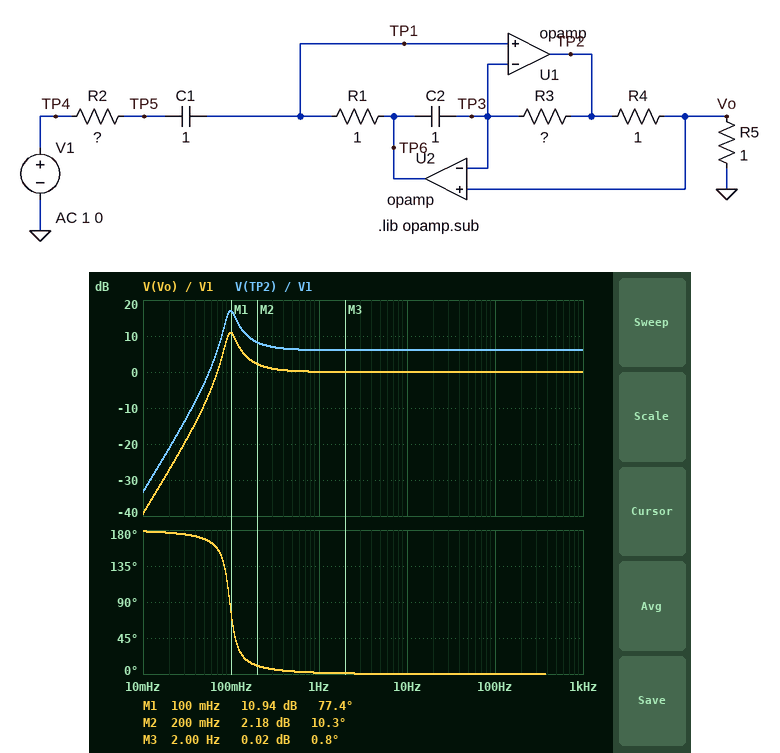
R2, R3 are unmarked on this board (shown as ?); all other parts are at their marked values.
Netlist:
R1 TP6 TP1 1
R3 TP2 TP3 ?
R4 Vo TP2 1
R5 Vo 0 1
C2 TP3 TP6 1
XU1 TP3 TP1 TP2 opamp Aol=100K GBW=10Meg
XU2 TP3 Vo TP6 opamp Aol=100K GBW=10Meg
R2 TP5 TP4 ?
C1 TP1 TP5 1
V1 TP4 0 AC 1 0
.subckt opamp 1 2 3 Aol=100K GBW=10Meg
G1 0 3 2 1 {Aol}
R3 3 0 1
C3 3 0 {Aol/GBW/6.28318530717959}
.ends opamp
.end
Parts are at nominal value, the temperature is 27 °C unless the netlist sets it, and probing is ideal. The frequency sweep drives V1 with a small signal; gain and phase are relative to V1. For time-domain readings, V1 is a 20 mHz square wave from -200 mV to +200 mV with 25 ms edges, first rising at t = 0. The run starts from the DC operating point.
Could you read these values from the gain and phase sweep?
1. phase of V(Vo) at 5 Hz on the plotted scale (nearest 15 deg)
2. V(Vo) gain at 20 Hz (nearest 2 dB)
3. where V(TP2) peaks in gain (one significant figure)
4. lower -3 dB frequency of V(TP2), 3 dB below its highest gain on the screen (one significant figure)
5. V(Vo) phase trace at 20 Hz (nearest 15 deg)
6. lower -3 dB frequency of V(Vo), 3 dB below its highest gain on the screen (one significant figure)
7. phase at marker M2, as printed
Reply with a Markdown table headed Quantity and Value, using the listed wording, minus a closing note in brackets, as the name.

| Quantity | Value |
|---|---|
| phase of V(Vo) at 5 Hz on the plotted scale | 0 deg |
| V(Vo) gain at 20 Hz | 0 dB |
| where V(TP2) peaks in gain | 100 mHz |
| lower -3 dB frequency of V(TP2), 3 dB below its highest gain on the screen | 90 mHz |
| V(Vo) phase trace at 20 Hz | 0 deg |
| lower -3 dB frequency of V(Vo), 3 dB below its highest gain on the screen | 90 mHz |
| phase at marker M2, as printed | 10.3 deg |
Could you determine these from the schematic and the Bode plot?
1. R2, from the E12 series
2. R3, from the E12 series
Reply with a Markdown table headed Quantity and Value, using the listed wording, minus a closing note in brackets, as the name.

| Quantity | Value |
|---|---|
| R2, from the E12 series | 0.47 Ω |
| R3, from the E12 series | 2.7 Ω |
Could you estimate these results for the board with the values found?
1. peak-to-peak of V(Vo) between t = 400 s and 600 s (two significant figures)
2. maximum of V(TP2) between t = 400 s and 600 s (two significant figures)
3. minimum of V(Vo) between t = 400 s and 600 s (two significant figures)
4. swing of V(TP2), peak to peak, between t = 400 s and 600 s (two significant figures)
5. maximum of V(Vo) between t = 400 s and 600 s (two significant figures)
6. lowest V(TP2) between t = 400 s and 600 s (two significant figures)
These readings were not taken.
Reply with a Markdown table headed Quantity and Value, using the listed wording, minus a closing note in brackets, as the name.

| Quantity | Value |
|---|---|
| peak-to-peak of V(Vo) between t = 400 s and 600 s | 880 mV |
| maximum of V(TP2) between t = 400 s and 600 s | 880 mV |
| minimum of V(Vo) between t = 400 s and 600 s | -440 mV |
| swing of V(TP2), peak to peak, between t = 400 s and 600 s | 1.8 V |
| maximum of V(Vo) between t = 400 s and 600 s | 440 mV |
| lowest V(TP2) between t = 400 s and 600 s | -880 mV |
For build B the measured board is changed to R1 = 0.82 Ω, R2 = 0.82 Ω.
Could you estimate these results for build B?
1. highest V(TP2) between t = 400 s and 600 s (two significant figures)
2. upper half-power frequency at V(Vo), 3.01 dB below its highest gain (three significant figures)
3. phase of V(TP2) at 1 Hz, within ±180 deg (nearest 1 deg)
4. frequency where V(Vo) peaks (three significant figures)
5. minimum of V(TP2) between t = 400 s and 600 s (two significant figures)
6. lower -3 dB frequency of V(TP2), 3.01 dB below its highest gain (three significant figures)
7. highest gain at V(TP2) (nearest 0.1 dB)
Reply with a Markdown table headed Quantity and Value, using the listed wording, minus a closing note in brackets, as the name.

| Quantity | Value |
|---|---|
| highest V(TP2) between t = 400 s and 600 s | 800 mV |
| upper half-power frequency at V(Vo), 3.01 dB below its highest gain | 190 mHz |
| phase of V(TP2) at 1 Hz, within ±180 deg | 3 deg |
| frequency where V(Vo) peaks | 116 mHz |
| minimum of V(TP2) between t = 400 s and 600 s | -800 mV |
| lower -3 dB frequency of V(TP2), 3.01 dB below its highest gain | 91.1 mHz |
| highest gain at V(TP2) | 11.5 dB |
